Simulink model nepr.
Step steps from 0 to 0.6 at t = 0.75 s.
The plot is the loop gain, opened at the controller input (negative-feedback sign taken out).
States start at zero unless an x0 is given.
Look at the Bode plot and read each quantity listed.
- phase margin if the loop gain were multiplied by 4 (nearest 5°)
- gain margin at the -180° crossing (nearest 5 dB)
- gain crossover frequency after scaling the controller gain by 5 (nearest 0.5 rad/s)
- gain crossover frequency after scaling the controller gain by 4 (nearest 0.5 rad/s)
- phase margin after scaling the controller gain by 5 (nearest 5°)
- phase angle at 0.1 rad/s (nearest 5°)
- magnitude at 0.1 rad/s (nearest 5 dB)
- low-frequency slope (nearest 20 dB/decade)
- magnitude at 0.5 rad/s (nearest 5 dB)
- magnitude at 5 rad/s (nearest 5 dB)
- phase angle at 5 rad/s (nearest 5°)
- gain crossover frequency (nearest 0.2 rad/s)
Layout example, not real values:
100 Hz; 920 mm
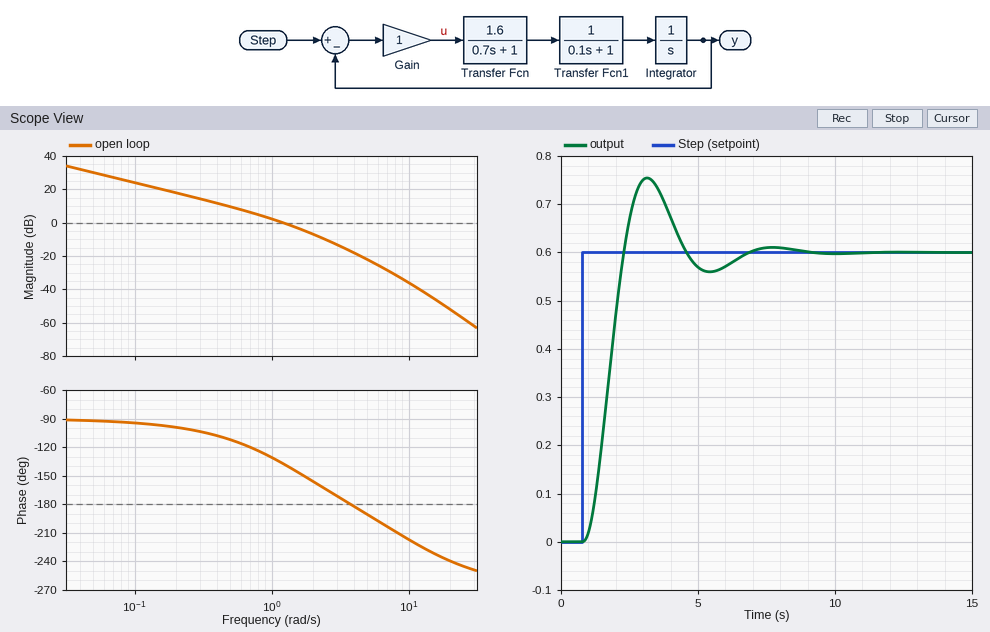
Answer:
10°; 15 dB; 3.0 rad/s; 3.0 rad/s; 5°; -95°; 25 dB; -20 dB/decade; 10 dB; -20 dB; -190°; 1.2 rad/s
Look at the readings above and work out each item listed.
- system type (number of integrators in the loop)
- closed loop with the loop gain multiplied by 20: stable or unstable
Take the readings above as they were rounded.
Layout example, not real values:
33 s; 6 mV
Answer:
1; unstable
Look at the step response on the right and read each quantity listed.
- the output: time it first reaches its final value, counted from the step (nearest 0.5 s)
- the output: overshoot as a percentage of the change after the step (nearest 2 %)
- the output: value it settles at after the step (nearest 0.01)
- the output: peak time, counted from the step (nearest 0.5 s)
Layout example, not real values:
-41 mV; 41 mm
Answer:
1.5 s; 26 %; 0.60; 2.5 s
